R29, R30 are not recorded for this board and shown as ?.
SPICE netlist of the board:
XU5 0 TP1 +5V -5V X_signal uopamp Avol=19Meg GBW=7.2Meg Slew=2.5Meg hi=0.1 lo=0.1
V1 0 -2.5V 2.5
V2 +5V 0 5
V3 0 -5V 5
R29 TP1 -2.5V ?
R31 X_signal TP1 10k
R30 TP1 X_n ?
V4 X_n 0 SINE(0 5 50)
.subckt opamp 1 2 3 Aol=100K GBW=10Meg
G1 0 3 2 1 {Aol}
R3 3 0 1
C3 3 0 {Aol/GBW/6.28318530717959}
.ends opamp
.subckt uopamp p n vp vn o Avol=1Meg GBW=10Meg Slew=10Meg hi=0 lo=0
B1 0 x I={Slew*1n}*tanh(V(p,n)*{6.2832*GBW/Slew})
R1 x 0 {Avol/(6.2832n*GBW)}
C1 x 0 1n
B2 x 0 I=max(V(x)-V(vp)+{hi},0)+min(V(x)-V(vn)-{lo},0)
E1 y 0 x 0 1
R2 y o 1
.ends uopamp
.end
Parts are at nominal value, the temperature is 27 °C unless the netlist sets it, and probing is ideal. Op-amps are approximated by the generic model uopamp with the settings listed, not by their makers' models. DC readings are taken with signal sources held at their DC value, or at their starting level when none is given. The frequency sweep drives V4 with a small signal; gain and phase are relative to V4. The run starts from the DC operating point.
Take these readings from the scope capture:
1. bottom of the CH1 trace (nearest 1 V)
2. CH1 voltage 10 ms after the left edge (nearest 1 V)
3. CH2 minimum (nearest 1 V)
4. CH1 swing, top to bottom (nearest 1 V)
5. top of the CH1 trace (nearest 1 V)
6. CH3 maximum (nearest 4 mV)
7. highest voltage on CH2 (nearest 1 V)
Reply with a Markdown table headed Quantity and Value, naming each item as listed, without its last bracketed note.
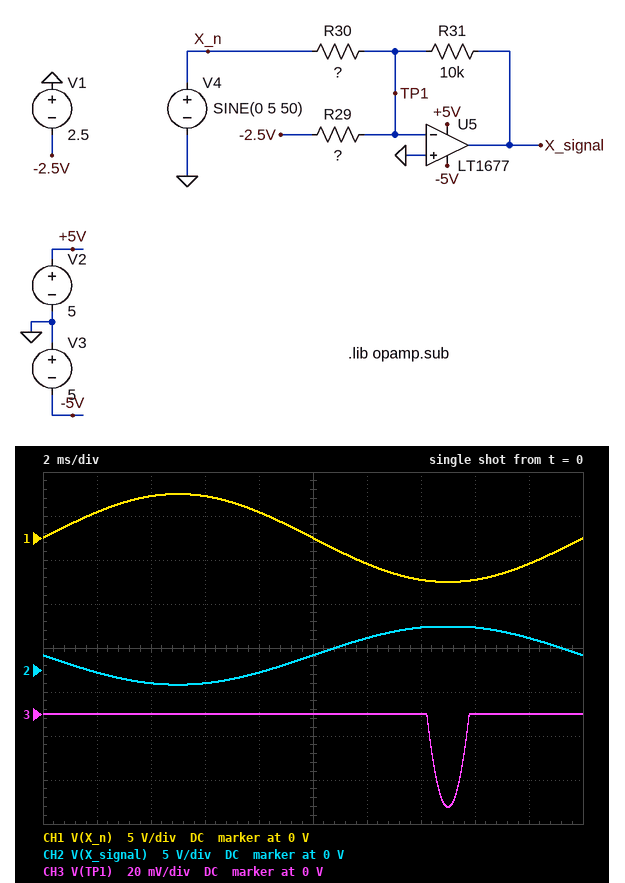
| Quantity | Value |
|---|---|
| bottom of the CH1 trace | -5 V |
| CH1 voltage 10 ms after the left edge | 0 V |
| CH2 minimum | -2 V |
| CH1 swing, top to bottom | 10 V |
| top of the CH1 trace | 5 V |
| CH3 maximum | 0 V |
| highest voltage on CH2 | 5 V |
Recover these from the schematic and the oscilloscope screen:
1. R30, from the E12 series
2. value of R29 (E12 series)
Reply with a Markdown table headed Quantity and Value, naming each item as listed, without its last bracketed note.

| Quantity | Value |
|---|---|
| R30, from the E12 series | 15 kΩ |
| value of R29 | 15 kΩ |
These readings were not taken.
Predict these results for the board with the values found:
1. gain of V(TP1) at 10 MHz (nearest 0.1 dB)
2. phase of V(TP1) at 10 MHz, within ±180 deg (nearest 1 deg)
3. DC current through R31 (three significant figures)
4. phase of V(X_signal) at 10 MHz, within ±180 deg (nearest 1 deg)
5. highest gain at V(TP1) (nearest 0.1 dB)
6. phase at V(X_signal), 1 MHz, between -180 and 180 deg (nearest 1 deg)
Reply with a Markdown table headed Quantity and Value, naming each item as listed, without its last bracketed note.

| Quantity | Value |
|---|---|
| gain of V(TP1) at 10 MHz | -11.3 dB |
| phase of V(TP1) at 10 MHz, within ±180 deg | 17 deg |
| DC current through R31 | 167 µA |
| phase of V(X_signal) at 10 MHz, within ±180 deg | 107 deg |
| highest gain at V(TP1) | -10.9 dB |
| phase at V(X_signal), 1 MHz, between -180 and 180 deg | 162 deg |
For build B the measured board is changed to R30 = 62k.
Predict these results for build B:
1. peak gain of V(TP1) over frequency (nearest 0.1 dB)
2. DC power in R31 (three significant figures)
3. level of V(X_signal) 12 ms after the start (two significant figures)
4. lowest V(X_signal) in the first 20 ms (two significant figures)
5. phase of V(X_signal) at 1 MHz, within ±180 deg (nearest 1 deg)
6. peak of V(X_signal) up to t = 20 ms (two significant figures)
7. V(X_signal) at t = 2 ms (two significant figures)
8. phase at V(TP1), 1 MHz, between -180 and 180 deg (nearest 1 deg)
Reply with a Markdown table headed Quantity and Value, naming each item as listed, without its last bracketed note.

| Quantity | Value |
|---|---|
| peak gain of V(TP1) over frequency | -21.1 dB |
| DC power in R31 | 278 µW |
| level of V(X_signal) 12 ms after the start | 2.1 V |
| lowest V(X_signal) in the first 20 ms | 860 mV |
| phase of V(X_signal) at 1 MHz, within ±180 deg | 166 deg |
| peak of V(X_signal) up to t = 20 ms | 2.5 V |
| V(X_signal) at t = 2 ms | 1.2 V |
| phase at V(TP1), 1 MHz, between -180 and 180 deg | 76 deg |
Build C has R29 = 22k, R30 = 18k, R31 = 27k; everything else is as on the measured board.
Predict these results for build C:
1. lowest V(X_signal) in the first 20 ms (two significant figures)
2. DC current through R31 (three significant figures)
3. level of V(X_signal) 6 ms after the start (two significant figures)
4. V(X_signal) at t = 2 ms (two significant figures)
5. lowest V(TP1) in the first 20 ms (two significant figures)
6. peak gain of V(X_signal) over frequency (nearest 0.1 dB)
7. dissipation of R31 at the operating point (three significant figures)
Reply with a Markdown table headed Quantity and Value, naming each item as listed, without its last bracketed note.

| Quantity | Value |
|---|---|
| lowest V(X_signal) in the first 20 ms | -4.4 V |
| DC current through R31 | 114 µA |
| level of V(X_signal) 6 ms after the start | -4.1 V |
| V(X_signal) at t = 2 ms | -1.3 V |
| lowest V(TP1) in the first 20 ms | -1.5 V |
| peak gain of V(X_signal) over frequency | 3.5 dB |
| dissipation of R31 at the operating point | 349 µW |
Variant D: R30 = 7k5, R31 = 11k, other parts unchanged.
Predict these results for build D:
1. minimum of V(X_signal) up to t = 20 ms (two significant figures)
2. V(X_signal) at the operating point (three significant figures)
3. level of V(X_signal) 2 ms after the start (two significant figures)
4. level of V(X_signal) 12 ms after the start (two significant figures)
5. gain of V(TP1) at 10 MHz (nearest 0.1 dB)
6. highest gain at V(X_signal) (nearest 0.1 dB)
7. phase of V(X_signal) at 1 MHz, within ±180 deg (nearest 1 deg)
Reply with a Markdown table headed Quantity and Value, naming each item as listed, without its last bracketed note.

| Quantity | Value |
|---|---|
| minimum of V(X_signal) up to t = 20 ms | -4.9 V |
| V(X_signal) at the operating point | 1.83 V |
| level of V(X_signal) 2 ms after the start | -2.5 V |
| level of V(X_signal) 12 ms after the start | 4.9 V |
| gain of V(TP1) at 10 MHz | -7.0 dB |
| highest gain at V(X_signal) | 3.3 dB |
| phase of V(X_signal) at 1 MHz, within ±180 deg | 156 deg |
